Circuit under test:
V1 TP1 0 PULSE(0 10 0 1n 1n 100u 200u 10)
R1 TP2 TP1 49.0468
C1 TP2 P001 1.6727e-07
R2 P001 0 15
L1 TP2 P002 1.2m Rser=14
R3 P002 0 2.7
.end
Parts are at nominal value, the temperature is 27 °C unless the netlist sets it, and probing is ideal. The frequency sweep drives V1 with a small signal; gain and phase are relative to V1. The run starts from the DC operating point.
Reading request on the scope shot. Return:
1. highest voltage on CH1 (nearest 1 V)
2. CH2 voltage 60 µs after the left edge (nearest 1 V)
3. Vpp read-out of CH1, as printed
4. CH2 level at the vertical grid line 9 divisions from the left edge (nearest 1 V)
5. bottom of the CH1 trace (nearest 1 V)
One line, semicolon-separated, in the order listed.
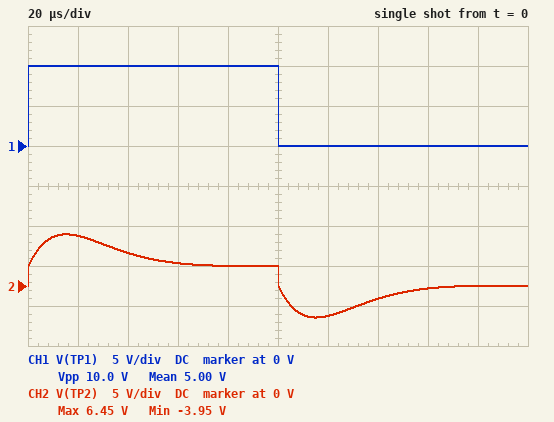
10 V; 3 V; 10.0 V; 0 V; 0 V
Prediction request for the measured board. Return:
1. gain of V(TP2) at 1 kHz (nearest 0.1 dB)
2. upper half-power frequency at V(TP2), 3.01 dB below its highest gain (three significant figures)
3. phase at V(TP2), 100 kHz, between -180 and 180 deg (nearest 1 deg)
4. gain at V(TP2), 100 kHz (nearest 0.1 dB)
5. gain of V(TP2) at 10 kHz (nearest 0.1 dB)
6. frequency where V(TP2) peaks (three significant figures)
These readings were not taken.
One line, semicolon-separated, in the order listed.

-11.1 dB; 25.3 kHz; -23 deg; -11.2 dB; -1.7 dB; 11.3 kHz
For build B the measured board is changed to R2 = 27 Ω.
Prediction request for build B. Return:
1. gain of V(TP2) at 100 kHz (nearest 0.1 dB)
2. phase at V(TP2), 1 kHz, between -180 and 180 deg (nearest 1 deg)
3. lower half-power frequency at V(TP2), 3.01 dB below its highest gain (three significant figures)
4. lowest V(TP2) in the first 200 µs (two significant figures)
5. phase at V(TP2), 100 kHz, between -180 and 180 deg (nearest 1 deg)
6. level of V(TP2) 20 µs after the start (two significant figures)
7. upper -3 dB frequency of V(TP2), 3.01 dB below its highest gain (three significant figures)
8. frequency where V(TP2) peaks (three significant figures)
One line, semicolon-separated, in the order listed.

-8.5 dB; 17 deg; 4.69 kHz; -3.7 V; -11 deg; 6.0 V; 26.9 kHz; 10.8 kHz
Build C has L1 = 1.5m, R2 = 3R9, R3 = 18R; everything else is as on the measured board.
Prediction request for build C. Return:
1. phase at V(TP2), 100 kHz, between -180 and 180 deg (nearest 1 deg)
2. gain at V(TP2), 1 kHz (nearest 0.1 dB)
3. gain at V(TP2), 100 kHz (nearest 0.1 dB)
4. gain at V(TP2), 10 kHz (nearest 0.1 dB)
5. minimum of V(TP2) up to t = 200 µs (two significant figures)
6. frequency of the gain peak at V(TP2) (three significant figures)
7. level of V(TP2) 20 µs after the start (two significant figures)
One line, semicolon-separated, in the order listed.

-57 deg; -7.7 dB; -14.3 dB; -1.4 dB; -3.3 V; 11.7 kHz; 7.2 V
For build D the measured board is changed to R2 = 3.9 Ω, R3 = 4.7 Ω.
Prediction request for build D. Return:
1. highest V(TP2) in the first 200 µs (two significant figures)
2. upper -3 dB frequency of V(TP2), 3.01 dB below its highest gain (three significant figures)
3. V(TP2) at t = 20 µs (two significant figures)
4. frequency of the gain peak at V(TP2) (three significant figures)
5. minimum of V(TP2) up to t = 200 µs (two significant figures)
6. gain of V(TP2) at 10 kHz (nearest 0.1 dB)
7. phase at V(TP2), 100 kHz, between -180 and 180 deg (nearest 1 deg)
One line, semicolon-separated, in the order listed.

6.9 V; 26.6 kHz; 6.7 V; 12.4 kHz; -4.1 V; -1.4 dB; -57 deg
